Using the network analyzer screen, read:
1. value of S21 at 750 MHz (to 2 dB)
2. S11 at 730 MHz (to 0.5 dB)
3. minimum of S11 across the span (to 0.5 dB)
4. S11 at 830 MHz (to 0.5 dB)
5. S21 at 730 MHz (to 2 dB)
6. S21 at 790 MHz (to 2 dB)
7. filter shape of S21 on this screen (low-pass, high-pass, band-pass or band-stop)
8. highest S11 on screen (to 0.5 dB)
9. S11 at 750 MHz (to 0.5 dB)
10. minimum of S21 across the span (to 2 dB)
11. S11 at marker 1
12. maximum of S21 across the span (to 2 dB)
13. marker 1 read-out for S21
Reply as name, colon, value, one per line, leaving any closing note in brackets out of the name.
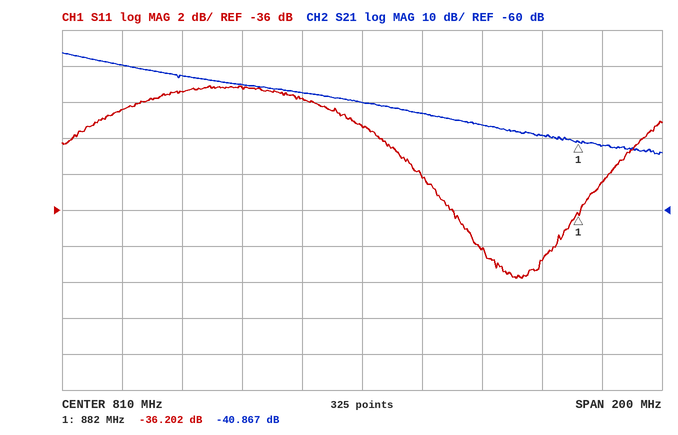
value of S21 at 750 MHz: -22 dB
S11 at 730 MHz: -30.5 dB
minimum of S11 across the span: -40.0 dB
S11 at 830 MHz: -34.0 dB
S21 at 730 MHz: -20 dB
S21 at 790 MHz: -28 dB
filter shape of S21 on this screen: low-pass
highest S11 on screen: -29.0 dB
S11 at 750 MHz: -29.5 dB
minimum of S21 across the span: -44 dB
S11 at marker 1: -36.202 dB
maximum of S21 across the span: -16 dB
marker 1 read-out for S21: -40.867 dB
